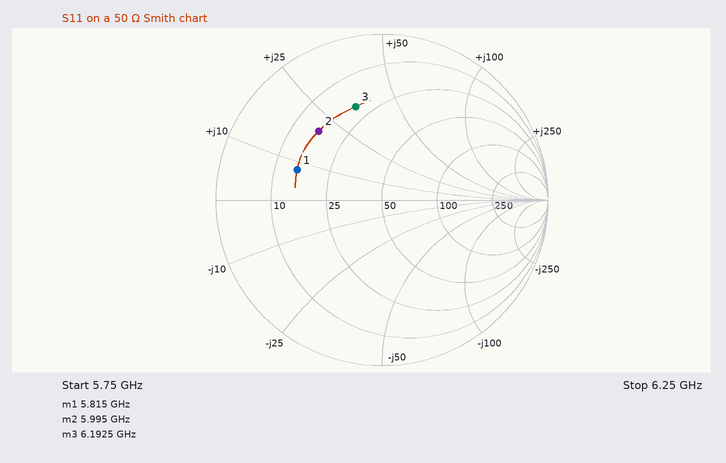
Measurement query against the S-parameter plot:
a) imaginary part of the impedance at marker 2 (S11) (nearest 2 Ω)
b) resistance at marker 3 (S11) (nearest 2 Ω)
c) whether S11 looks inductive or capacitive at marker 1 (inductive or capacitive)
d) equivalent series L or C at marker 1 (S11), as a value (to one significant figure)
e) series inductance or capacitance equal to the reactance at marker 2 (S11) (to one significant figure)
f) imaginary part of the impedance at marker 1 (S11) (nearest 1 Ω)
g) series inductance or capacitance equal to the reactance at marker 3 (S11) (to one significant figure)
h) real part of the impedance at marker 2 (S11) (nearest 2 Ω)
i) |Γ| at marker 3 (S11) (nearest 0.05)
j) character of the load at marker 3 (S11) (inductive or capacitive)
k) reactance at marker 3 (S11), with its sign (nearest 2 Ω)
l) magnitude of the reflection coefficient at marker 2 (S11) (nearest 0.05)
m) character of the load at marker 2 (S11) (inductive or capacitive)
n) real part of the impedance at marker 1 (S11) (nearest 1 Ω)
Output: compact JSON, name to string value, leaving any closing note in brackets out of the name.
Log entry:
{"imaginary part of the impedance at marker 2 (S11)": "+20 Ω", "resistance at marker 3 (S11)": "20 Ω", "whether S11 looks inductive or capacitive at marker 1": "inductive", "equivalent series L or C at marker 1 (S11), as a value": "200 pH", "series inductance or capacitance equal to the reactance at marker 2 (S11)": "500 pH", "imaginary part of the impedance at marker 1 (S11)": "+8 Ω", "series inductance or capacitance equal to the reactance at marker 3 (S11)": "900 pH", "real part of the impedance at marker 2 (S11)": "16 Ω", "|Γ| at marker 3 (S11)": "0.60", "character of the load at marker 3 (S11)": "inductive", "reactance at marker 3 (S11), with its sign": "+34 Ω", "magnitude of the reflection coefficient at marker 2 (S11)": "0.55", "character of the load at marker 2 (S11)": "inductive", "real part of the impedance at marker 1 (S11)": "15 Ω"}
